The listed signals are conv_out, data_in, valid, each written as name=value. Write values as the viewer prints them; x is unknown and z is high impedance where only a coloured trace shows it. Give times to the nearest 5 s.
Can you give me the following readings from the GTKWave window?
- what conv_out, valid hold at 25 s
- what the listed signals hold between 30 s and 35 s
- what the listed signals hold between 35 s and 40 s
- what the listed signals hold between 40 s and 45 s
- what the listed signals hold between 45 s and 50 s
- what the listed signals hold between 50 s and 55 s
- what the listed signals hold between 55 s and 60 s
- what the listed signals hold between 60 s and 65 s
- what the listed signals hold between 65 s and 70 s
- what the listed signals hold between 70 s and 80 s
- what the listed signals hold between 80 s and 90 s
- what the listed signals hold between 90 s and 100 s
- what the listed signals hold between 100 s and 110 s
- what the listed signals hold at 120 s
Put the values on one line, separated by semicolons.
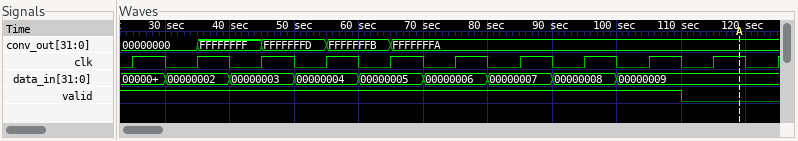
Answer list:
conv_out=00000000, valid=1; conv_out=00000000, data_in=00000002, valid=1; conv_out=FFFFFFFF, data_in=00000002, valid=1; conv_out=FFFFFFFF, data_in=00000003, valid=1; conv_out=FFFFFFFD, data_in=00000003, valid=1; conv_out=FFFFFFFD, data_in=00000004, valid=1; conv_out=FFFFFFFB, data_in=00000004, valid=1; conv_out=FFFFFFFB, data_in=00000005, valid=1; conv_out=FFFFFFFA, data_in=00000005, valid=1; conv_out=FFFFFFFA, data_in=00000006, valid=1; conv_out=FFFFFFFA, data_in=00000007, valid=1; conv_out=FFFFFFFA, data_in=00000008, valid=1; conv_out=FFFFFFFA, data_in=00000009, valid=1; conv_out=FFFFFFFA, data_in=00000009, valid=0
